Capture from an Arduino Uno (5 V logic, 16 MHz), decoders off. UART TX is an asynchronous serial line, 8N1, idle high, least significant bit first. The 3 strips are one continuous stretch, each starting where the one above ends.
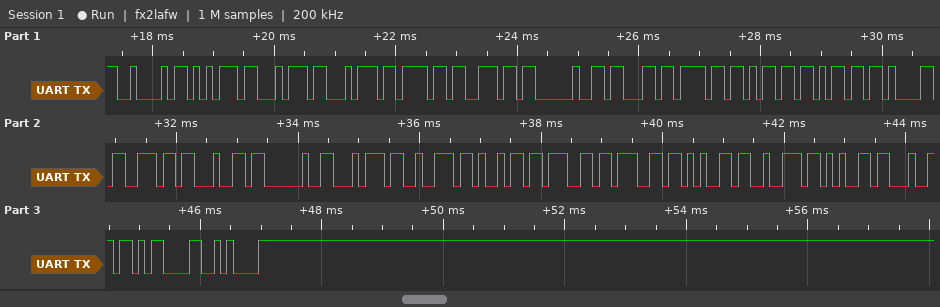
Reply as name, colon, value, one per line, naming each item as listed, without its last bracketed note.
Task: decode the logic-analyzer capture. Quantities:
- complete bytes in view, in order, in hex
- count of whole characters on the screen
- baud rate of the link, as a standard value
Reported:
complete bytes in view, in order, in hex: 42 75 74 74 6F 6E 20 63 6F 6D 6D 61 6E 64 20 74 72 69 67 67 65 72 65 64 0D 0A
count of whole characters on the screen: 26
baud rate of the link, as a standard value: 9600 baud
